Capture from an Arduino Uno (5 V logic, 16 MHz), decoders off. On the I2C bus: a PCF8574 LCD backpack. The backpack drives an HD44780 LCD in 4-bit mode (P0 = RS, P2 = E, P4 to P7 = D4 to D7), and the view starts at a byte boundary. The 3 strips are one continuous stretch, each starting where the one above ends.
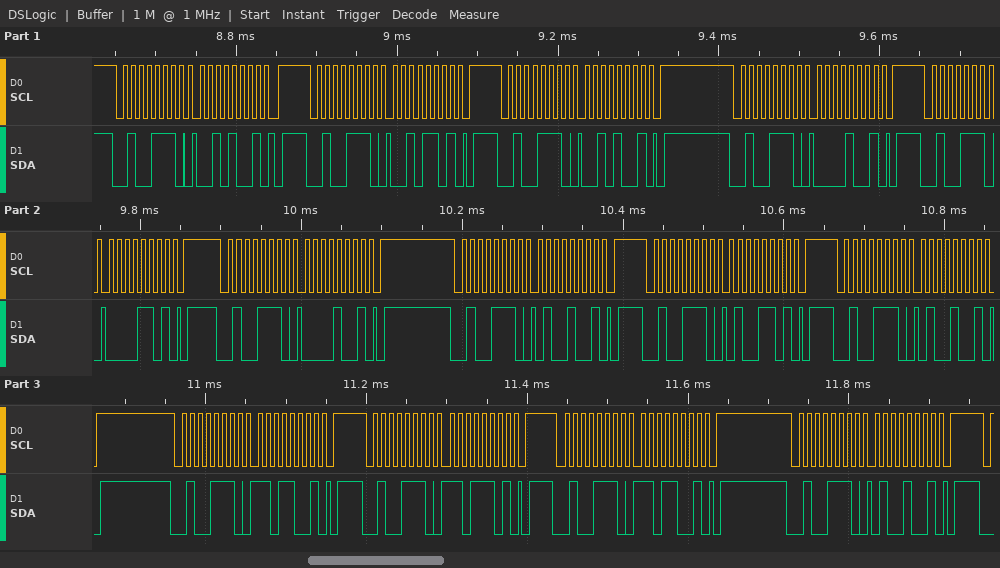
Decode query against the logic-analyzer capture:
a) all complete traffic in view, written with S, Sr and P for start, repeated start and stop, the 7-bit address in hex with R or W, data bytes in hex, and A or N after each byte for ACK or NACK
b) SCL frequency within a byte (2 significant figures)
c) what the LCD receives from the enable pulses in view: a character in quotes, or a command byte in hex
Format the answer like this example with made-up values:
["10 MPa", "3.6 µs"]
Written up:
["S 27W A 29 A P S 27W A 2D A P S 27W A 29 A P S 27W A 09 A P S 27W A 0D A P S 27W A 09 A P S 27W A 49 A P S 27W A 4D A P S 27W A 49 A P S 27W A D9 A P S 27W A DD A P S 27W A D9 A P S 27W A 49 A P", "100 kHz", "' ' 'M'"]
